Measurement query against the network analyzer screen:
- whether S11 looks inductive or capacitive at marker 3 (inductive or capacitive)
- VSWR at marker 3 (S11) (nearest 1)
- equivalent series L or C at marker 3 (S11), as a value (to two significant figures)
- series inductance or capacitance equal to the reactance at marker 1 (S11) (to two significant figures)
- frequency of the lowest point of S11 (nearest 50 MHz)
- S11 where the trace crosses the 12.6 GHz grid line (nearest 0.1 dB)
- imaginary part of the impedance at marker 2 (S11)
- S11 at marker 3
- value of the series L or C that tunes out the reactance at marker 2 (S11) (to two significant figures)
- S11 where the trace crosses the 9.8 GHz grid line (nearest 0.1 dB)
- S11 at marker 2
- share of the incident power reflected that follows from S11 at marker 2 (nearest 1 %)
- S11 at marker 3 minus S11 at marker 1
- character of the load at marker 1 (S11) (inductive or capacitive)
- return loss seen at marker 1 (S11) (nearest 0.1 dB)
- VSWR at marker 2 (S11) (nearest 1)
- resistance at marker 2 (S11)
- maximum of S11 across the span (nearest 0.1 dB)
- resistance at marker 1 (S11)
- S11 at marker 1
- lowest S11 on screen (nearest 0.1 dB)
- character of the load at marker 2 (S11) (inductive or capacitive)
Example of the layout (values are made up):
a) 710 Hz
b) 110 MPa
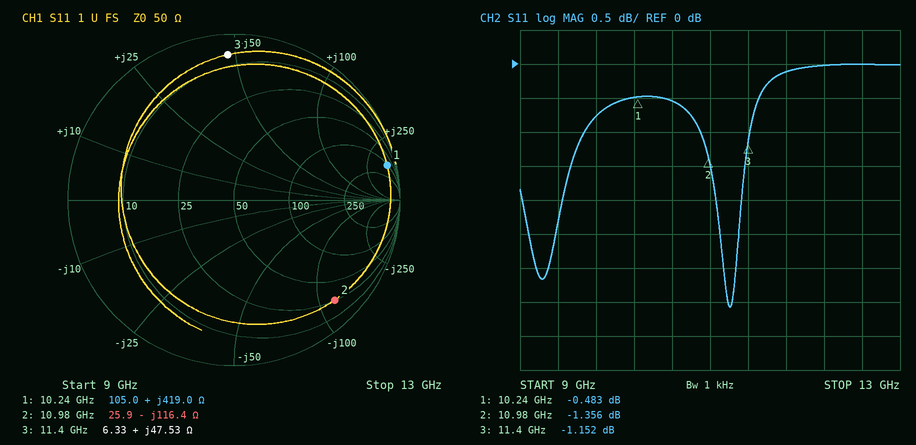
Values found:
a) inductive
b) 15
c) 660 pH
d) 6.5 nH
e) 11.20 GHz
f) 0.0 dB
g) -116.4 Ω
h) -1.152 dB
i) 1.7 nH
j) -0.8 dB
k) -1.356 dB
l) 73 %
m) -0.669 dB
n) inductive
o) 0.5 dB
p) 13
q) 25.9 Ω
r) 0.0 dB
s) 105.0 Ω
t) -0.483 dB
u) -3.6 dB
v) capacitive
